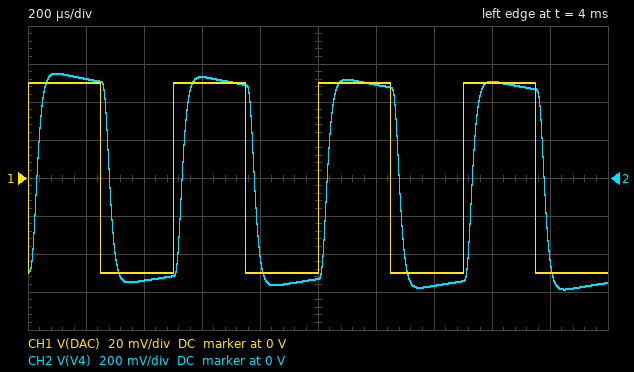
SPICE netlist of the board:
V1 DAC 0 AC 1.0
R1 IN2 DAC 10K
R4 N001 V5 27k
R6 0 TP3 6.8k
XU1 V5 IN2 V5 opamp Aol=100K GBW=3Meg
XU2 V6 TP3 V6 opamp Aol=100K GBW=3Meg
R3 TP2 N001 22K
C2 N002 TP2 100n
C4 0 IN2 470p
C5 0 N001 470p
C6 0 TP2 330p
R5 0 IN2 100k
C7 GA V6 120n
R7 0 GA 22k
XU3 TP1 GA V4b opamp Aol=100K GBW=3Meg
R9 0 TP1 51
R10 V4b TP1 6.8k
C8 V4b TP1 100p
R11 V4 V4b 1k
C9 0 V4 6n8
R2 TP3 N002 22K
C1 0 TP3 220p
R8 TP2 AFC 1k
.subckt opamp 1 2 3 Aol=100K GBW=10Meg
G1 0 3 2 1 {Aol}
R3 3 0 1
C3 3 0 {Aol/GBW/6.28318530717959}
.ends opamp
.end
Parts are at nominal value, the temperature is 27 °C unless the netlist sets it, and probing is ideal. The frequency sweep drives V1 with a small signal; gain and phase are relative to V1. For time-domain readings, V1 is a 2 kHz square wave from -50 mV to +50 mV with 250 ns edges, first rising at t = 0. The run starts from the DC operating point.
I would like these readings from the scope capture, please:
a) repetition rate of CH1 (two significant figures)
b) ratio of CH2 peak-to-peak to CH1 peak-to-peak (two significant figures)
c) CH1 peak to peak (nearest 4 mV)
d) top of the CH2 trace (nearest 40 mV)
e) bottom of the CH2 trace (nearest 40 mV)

2.0 kHz
11
100 mV
560 mV
-600 mV
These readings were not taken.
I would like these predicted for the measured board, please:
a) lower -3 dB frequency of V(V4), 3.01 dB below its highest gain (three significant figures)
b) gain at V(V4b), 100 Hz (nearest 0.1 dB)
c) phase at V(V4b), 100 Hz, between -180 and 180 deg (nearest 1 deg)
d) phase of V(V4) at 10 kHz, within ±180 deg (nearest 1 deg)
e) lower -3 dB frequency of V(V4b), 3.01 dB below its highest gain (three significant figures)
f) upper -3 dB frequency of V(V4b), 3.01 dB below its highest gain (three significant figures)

65.5 Hz
19.0 dB
42 deg
-115 deg
65.6 Hz
9.72 kHz
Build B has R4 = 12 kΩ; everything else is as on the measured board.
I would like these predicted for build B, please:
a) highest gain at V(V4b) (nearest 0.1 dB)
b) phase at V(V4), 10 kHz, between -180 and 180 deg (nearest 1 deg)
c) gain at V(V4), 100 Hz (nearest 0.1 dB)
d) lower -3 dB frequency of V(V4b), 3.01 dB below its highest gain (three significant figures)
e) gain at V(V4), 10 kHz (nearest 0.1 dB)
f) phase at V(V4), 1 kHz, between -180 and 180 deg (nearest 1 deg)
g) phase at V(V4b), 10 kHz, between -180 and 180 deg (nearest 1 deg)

22.4 dB
-102 deg
20.8 dB
68.4 Hz
19.5 dB
-6 deg
-79 deg
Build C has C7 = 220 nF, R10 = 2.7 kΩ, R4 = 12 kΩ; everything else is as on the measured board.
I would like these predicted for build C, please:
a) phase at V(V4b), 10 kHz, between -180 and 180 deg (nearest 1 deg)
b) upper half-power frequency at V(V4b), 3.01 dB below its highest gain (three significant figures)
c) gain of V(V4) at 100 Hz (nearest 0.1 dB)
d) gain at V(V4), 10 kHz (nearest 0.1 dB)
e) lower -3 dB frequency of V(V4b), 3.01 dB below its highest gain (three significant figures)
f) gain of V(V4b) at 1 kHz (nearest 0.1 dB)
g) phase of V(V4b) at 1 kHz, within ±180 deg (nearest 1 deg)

-64 deg
15.1 kHz
13.8 dB
12.3 dB
45.2 Hz
14.5 dB
-3 deg
